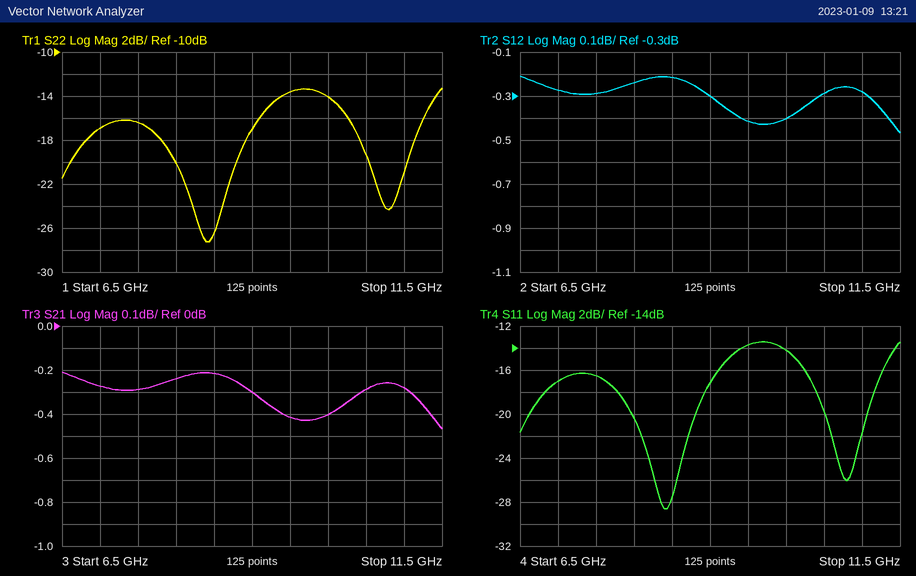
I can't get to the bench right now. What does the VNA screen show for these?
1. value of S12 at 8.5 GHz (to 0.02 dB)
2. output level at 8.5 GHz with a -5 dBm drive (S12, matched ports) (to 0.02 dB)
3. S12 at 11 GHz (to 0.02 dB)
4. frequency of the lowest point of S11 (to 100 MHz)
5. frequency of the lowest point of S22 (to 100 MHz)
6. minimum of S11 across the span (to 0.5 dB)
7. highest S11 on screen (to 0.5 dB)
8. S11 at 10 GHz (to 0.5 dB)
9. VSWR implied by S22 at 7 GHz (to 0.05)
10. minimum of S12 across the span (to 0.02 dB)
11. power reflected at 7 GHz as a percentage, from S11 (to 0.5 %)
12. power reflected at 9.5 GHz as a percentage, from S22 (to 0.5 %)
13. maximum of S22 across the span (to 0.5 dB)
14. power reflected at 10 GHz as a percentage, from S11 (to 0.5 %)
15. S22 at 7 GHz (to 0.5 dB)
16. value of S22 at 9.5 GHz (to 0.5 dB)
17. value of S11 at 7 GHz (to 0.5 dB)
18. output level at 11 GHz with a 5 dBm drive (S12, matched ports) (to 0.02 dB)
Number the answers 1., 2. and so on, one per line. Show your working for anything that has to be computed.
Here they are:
1. -0.22 dB
2. -5 dBm + (-0.22 dB) = -5.22 dBm
3. -0.28 dB
4. 8.4 GHz
5. 8.4 GHz
6. -28.5 dB
7. -13.5 dB
8. -14.0 dB
9. |Γ| = 10^(-17/20) = 0.1413; VSWR = (1 + 0.1413)/(1 − 0.1413) ≈ 1.33, so 1.35 to the nearest 0.05
10. -0.46 dB
11. 10^(-17/10) ≈ 2.0 %
12. 10^(-13.5/10) ≈ 4.5 %
13. -13.5 dB
14. 10^(-14/10) ≈ 4.0 %
15. -17.0 dB
16. -13.5 dB
17. -17.0 dB
18. 5 dBm + (-0.28 dB) = 4.72 dBm
